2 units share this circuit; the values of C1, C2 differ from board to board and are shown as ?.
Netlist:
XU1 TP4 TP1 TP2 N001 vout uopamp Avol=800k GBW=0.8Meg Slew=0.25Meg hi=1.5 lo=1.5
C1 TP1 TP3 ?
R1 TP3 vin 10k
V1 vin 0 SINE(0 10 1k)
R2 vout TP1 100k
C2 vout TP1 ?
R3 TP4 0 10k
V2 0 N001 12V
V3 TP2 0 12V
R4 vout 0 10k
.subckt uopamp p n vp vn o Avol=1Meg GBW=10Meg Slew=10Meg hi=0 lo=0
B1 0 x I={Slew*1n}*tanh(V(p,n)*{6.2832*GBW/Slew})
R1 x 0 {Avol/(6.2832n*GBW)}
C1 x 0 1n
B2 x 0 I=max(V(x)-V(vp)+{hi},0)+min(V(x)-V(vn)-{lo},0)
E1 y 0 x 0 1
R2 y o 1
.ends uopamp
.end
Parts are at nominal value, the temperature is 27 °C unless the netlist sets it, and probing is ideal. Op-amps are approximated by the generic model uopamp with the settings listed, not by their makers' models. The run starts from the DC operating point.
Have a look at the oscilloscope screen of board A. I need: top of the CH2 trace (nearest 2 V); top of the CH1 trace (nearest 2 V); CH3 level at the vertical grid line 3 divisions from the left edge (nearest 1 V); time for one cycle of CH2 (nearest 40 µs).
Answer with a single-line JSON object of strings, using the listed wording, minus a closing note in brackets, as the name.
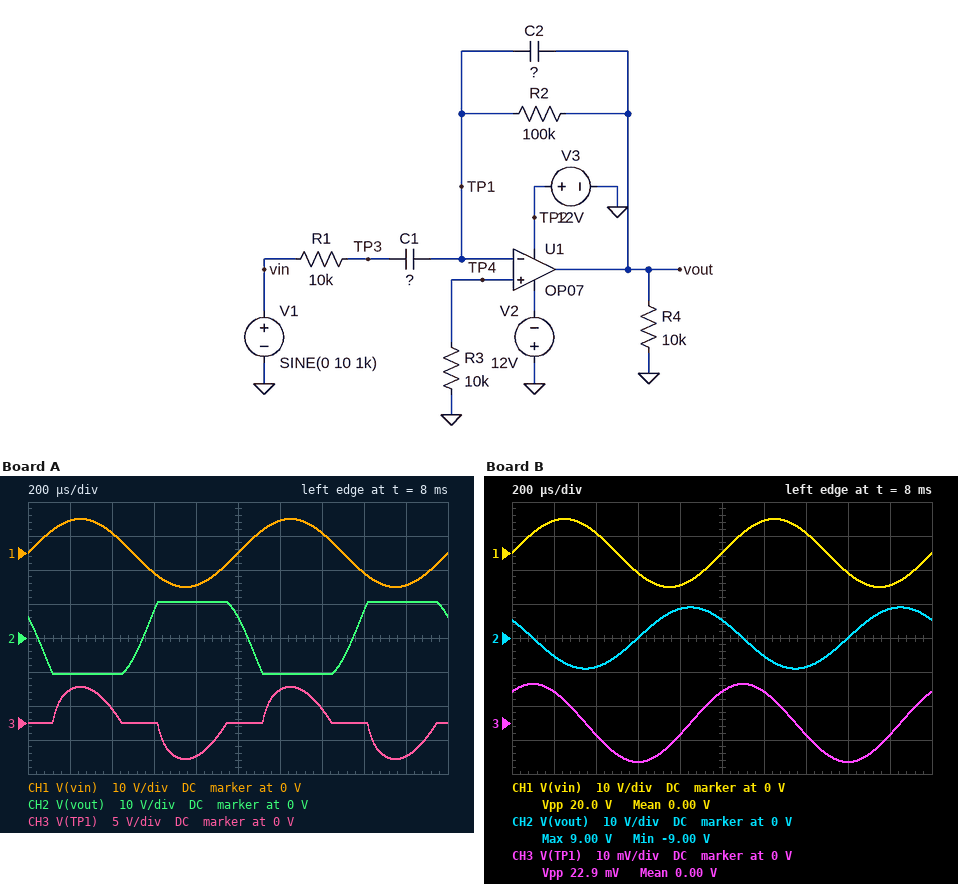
{"top of the CH2 trace": "10 V", "top of the CH1 trace": "10 V", "CH3 level at the vertical grid line 3 divisions from the left edge": "0 V", "time for one cycle of CH2": "1.00 ms"}
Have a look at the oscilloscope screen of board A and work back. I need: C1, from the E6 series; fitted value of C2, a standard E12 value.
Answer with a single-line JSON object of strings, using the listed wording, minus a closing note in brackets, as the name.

{"C1, from the E6 series": "15 nF", "fitted value of C2, a standard E12 value": "3.3 nF"}
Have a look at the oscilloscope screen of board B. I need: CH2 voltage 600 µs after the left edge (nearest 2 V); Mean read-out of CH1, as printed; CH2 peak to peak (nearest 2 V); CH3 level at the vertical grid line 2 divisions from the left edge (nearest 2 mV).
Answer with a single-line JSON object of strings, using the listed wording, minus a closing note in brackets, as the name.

{"CH2 voltage 600 µs after the left edge": "0 V", "Mean read-out of CH1, as printed": "0.00 V", "CH2 peak to peak": "18 V", "CH3 level at the vertical grid line 2 divisions from the left edge": "-4 mV"}
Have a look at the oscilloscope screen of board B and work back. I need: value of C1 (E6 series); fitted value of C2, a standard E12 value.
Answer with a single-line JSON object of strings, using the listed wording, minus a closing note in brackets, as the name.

{"value of C1": "15 nF", "fitted value of C2, a standard E12 value": "12 nF"}
